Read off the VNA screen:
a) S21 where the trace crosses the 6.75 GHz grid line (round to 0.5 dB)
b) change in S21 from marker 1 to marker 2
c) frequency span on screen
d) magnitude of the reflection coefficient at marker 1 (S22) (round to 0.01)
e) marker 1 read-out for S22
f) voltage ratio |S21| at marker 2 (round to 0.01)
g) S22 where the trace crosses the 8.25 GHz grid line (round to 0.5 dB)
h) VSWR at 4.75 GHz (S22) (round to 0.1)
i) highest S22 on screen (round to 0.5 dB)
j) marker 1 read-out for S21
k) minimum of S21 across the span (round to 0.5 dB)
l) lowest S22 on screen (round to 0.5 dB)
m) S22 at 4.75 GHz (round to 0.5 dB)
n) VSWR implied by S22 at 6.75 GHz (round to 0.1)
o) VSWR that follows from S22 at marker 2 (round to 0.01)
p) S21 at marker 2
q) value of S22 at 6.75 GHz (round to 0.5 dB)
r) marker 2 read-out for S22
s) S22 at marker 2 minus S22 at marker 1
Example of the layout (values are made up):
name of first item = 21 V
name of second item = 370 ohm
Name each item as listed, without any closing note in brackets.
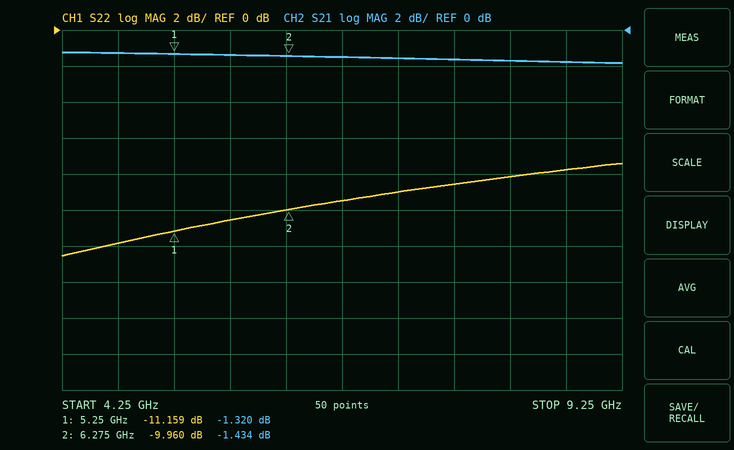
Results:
S21 where the trace crosses the 6.75 GHz grid line = -1.5 dB
change in S21 from marker 1 to marker 2 = -0.114 dB
frequency span on screen = 5 GHz
magnitude of the reflection coefficient at marker 1 (S22) = 0.28
marker 1 read-out for S22 = -11.159 dB
voltage ratio |S21| at marker 2 = 0.85
S22 where the trace crosses the 8.25 GHz grid line = -8.0 dB
VSWR at 4.75 GHz (S22) = 1.7
highest S22 on screen = -7.5 dB
marker 1 read-out for S21 = -1.320 dB
minimum of S21 across the span = -2.0 dB
lowest S22 on screen = -12.5 dB
S22 at 4.75 GHz = -12.0 dB
VSWR implied by S22 at 6.75 GHz = 2.0
VSWR that follows from S22 at marker 2 = 1.93
S21 at marker 2 = -1.434 dB
value of S22 at 6.75 GHz = -9.5 dB
marker 2 read-out for S22 = -9.960 dB
S22 at marker 2 minus S22 at marker 1 = 1.199 dB
